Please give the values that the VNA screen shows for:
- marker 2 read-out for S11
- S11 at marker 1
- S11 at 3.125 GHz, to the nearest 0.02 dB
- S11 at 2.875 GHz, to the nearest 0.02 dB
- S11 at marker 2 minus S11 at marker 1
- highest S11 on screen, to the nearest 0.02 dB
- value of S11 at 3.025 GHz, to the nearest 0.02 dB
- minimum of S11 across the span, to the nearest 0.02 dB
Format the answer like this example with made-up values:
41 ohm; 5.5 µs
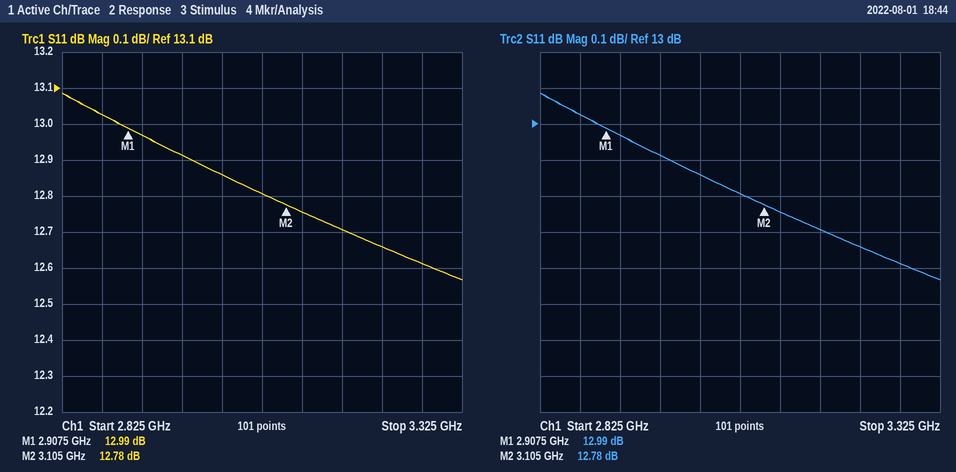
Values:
12.78 dB; 12.99 dB; 12.76 dB; 13.02 dB; -0.21 dB; 13.08 dB; 12.86 dB; 12.56 dB
